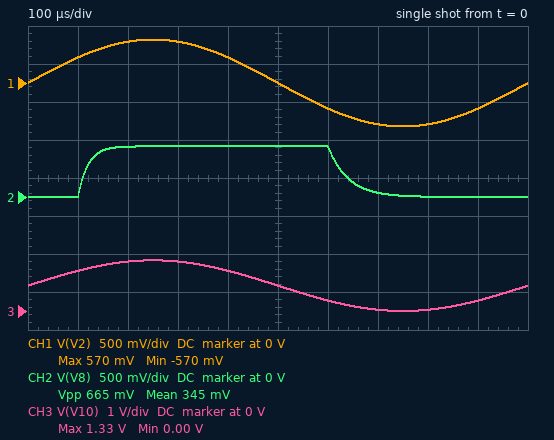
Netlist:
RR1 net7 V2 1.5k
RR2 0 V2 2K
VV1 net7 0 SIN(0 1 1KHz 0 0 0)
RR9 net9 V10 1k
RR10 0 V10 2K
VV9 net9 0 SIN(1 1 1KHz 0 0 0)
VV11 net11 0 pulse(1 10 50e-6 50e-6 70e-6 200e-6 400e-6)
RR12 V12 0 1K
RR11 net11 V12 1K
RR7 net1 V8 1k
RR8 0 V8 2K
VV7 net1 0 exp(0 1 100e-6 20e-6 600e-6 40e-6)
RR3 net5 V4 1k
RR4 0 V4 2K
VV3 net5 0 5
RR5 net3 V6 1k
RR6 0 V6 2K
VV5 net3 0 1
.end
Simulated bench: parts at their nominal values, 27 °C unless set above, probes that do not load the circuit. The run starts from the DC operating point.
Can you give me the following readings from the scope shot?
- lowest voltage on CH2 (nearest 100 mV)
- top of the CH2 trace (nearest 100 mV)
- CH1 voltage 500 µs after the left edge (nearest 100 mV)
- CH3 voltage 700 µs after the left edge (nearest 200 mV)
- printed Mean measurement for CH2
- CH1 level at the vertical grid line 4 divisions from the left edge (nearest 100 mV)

0 V
700 mV
0 V
0 V
345 mV
300 mV
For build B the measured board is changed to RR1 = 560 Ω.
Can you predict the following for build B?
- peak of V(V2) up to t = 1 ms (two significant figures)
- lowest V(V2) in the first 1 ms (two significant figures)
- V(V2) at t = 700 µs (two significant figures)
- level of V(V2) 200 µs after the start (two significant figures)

780 mV
-780 mV
-740 mV
740 mV
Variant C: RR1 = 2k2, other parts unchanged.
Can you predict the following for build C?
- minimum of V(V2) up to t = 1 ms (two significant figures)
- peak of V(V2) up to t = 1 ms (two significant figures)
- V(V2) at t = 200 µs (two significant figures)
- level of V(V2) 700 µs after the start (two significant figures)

-480 mV
480 mV
450 mV
-450 mV
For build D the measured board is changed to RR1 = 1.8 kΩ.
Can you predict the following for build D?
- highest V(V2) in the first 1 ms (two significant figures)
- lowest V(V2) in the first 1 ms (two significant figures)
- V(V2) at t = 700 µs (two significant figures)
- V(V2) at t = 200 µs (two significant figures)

530 mV
-530 mV
-500 mV
500 mV
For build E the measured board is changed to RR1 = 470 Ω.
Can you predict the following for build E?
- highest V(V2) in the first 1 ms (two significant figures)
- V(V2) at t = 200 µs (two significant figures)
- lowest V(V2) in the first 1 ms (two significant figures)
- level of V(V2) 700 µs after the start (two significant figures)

810 mV
770 mV
-810 mV
-770 mV
